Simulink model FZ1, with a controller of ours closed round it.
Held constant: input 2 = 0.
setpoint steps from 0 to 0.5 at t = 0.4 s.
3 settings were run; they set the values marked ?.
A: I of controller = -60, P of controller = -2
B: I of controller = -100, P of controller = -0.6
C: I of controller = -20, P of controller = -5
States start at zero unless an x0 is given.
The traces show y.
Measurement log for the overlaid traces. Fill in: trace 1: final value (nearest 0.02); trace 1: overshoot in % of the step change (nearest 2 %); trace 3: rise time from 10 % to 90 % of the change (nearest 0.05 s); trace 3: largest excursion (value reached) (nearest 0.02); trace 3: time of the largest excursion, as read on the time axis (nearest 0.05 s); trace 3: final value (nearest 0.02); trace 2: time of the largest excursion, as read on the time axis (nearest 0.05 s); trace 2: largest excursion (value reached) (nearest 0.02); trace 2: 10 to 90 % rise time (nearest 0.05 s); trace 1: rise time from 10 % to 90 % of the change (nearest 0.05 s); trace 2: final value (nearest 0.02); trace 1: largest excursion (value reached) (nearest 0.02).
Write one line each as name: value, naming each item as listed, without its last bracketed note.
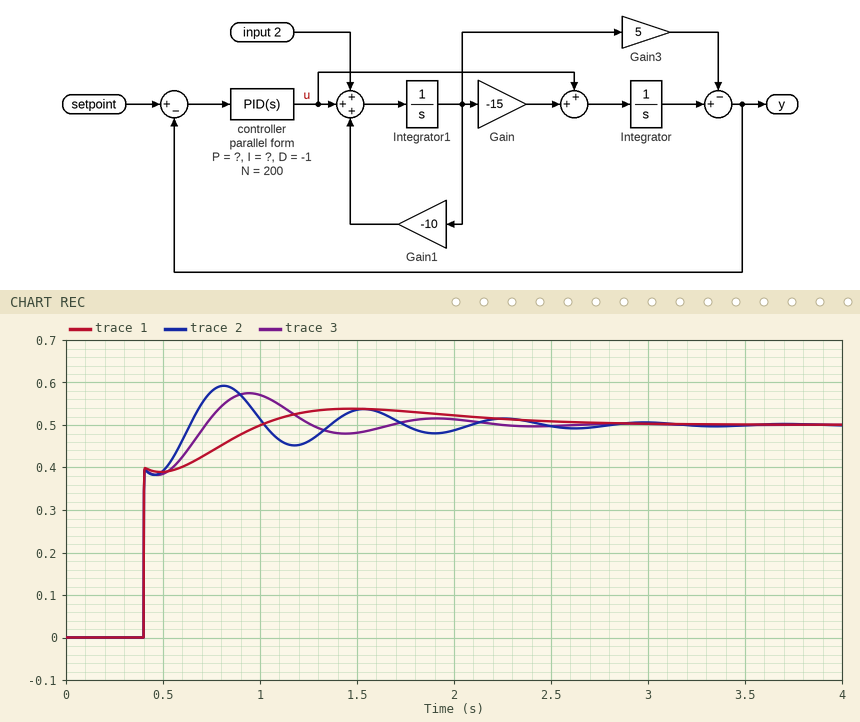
trace 1: final value: 0.50
trace 1: overshoot in % of the step change: 8 %
trace 3: rise time from 10 % to 90 % of the change: 0.25 s
trace 3: largest excursion (value reached): 0.58
trace 3: time of the largest excursion, as read on the time axis: 0.95 s
trace 3: final value: 0.50
trace 2: time of the largest excursion, as read on the time axis: 0.80 s
trace 2: largest excursion (value reached): 0.60
trace 2: 10 to 90 % rise time: 0.20 s
trace 1: rise time from 10 % to 90 % of the change: 0.40 s
trace 2: final value: 0.50
trace 1: largest excursion (value reached): 0.54
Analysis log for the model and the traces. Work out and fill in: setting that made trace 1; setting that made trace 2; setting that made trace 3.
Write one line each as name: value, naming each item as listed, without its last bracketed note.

setting that made trace 1: C
setting that made trace 2: B
setting that made trace 3: A
